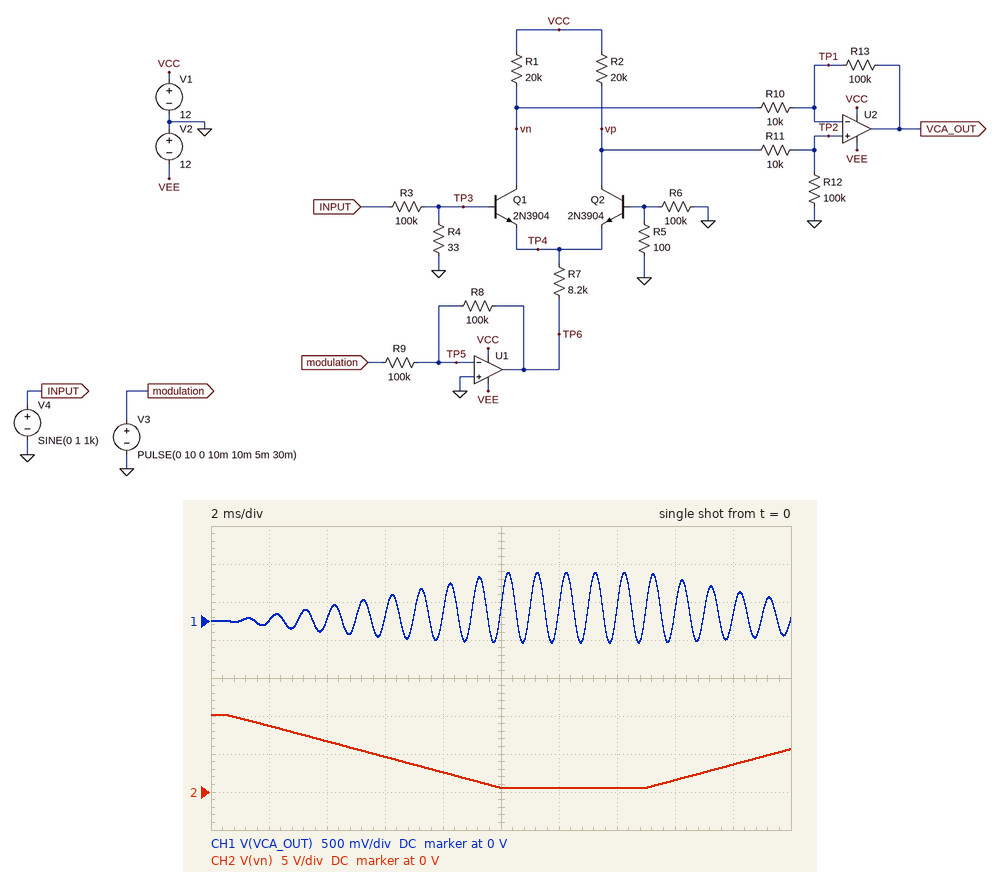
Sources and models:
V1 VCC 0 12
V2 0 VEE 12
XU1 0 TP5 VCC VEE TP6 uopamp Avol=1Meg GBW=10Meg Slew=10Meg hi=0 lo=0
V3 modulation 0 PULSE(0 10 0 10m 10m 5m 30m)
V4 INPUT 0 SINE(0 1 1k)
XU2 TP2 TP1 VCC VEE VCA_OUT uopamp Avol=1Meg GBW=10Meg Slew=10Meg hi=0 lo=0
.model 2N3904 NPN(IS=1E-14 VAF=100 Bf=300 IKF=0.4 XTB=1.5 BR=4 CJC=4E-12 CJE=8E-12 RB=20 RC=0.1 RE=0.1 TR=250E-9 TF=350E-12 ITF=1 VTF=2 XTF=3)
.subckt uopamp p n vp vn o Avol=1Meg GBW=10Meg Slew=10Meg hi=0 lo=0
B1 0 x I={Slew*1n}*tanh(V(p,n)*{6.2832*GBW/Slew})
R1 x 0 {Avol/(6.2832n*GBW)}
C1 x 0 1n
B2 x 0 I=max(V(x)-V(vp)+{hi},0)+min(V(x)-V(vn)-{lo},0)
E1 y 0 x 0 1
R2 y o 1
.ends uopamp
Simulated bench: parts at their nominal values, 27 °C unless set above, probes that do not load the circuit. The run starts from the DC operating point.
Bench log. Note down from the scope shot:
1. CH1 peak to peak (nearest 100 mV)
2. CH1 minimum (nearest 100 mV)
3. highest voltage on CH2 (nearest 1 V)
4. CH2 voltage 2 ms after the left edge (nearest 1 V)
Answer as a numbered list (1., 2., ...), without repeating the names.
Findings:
1. 900 mV
2. -300 mV
3. 10 V
4. 9 V
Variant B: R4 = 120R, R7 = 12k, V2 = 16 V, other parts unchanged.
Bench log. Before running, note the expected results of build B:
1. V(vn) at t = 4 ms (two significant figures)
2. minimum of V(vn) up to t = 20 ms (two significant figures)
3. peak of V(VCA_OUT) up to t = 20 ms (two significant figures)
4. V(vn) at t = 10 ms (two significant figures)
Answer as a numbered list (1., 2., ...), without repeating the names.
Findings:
1. 7.8 V
2. 3.5 V
3. 1.1 V
4. 3.6 V
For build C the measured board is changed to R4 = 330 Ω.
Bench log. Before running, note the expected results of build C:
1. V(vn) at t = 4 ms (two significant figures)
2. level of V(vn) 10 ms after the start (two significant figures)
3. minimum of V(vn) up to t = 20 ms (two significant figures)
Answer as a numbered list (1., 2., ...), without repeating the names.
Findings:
1. 6.7 V
2. 510 mV
3. 390 mV
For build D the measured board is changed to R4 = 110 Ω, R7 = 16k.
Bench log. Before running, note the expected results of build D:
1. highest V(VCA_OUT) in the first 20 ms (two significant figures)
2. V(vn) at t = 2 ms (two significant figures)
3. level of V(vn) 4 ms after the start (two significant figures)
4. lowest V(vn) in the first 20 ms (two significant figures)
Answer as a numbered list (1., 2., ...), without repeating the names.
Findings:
1. 800 mV
2. 9.4 V
3. 8.4 V
4. 5.2 V
